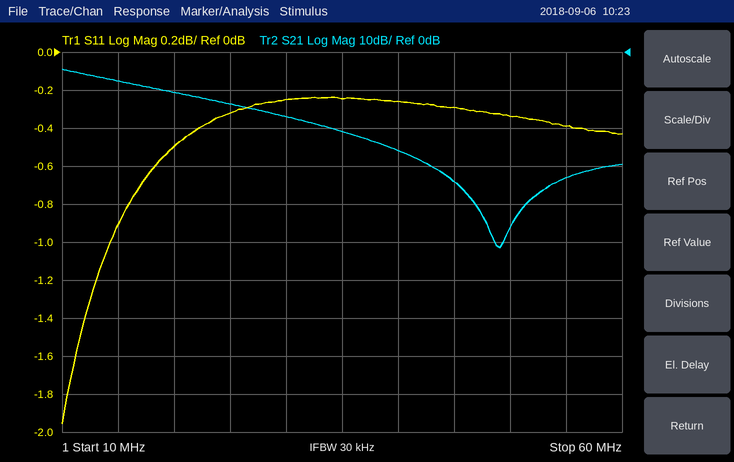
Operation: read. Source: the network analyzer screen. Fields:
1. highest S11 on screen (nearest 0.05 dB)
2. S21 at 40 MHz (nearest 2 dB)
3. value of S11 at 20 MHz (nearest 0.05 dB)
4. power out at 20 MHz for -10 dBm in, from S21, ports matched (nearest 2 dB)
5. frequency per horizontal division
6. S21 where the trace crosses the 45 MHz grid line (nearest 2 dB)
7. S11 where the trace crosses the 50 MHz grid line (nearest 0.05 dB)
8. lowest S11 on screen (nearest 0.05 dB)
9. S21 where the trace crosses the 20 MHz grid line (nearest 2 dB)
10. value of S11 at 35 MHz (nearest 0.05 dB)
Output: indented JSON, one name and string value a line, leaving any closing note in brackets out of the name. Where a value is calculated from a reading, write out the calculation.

{
  "highest S11 on screen": "-0.25 dB",
  "S21 at 40 MHz": "-26 dB",
  "value of S11 at 20 MHz": "-0.50 dB",
  "power out at 20 MHz for -10 dBm in, from S21, ports matched": "-10 dBm + (-10 dB) = -20 dBm",
  "frequency per horizontal division": "5 MHz",
  "S21 where the trace crosses the 45 MHz grid line": "-34 dB",
  "S11 where the trace crosses the 50 MHz grid line": "-0.35 dB",
  "lowest S11 on screen": "-1.95 dB",
  "S21 where the trace crosses the 20 MHz grid line": "-10 dB",
  "value of S11 at 35 MHz": "-0.25 dB"
}
